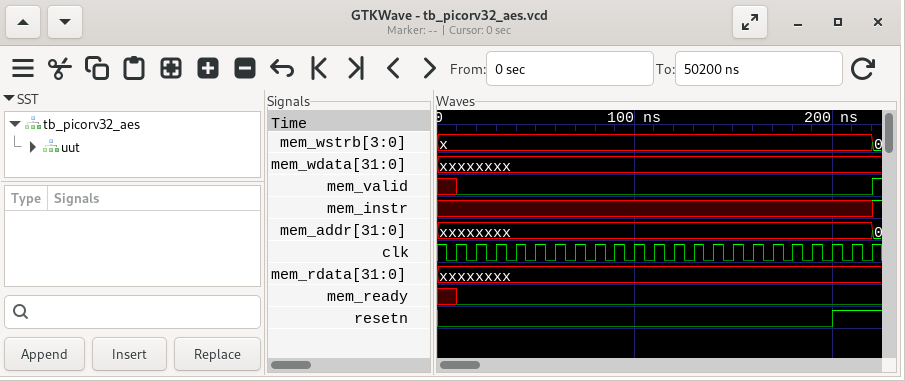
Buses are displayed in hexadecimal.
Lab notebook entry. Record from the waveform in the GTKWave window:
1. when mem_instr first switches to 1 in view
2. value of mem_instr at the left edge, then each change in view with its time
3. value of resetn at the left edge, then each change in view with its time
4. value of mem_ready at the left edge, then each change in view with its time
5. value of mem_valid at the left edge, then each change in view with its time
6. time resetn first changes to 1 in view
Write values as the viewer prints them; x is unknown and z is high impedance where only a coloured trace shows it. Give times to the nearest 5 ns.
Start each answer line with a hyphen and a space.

- 220 ns
- x, 1 at 220 ns
- 0, 1 at 200 ns
- x, 0 at 10 ns
- x, 0 at 10 ns, 1 at 220 ns
- 200 ns
